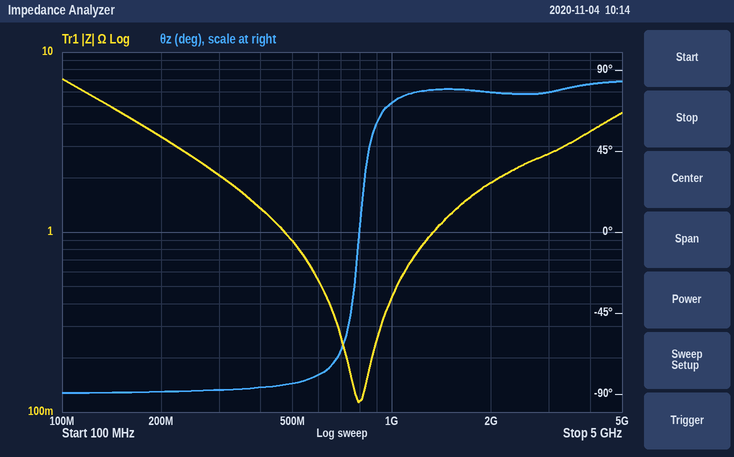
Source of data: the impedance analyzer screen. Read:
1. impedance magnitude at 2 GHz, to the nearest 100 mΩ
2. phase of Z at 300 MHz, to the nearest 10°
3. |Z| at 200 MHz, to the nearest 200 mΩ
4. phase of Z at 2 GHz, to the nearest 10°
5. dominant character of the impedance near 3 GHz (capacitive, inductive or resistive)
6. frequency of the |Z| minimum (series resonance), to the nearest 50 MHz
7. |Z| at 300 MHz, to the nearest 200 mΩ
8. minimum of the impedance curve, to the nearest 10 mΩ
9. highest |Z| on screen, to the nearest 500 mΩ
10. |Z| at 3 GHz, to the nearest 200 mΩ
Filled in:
1.9 Ω
-90°
3.4 Ω
80°
inductive
800 MHz
2.0 Ω
110 mΩ
7.0 Ω
2.8 Ω
